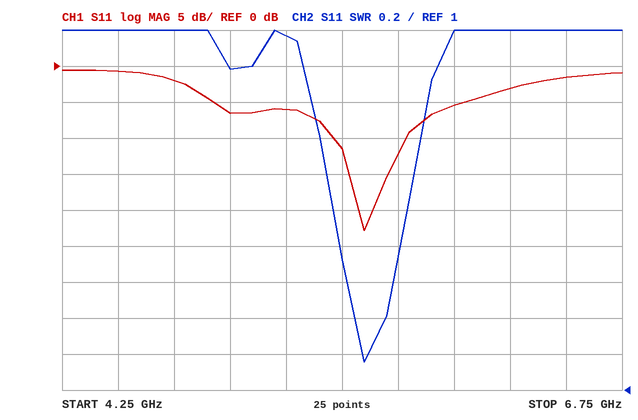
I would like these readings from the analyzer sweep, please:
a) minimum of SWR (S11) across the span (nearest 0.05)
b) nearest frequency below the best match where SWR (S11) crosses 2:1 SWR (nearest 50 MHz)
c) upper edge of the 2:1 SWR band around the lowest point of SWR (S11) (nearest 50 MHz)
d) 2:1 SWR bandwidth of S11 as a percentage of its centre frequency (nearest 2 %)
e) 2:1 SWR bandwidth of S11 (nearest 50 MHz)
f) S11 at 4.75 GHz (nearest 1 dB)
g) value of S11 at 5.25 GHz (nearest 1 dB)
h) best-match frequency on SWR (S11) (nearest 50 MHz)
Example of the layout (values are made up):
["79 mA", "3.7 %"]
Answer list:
["1.15", "5.45 GHz", "5.80 GHz", "6 %", "350 MHz", "-2 dB", "-6 dB", "5.60 GHz"]
